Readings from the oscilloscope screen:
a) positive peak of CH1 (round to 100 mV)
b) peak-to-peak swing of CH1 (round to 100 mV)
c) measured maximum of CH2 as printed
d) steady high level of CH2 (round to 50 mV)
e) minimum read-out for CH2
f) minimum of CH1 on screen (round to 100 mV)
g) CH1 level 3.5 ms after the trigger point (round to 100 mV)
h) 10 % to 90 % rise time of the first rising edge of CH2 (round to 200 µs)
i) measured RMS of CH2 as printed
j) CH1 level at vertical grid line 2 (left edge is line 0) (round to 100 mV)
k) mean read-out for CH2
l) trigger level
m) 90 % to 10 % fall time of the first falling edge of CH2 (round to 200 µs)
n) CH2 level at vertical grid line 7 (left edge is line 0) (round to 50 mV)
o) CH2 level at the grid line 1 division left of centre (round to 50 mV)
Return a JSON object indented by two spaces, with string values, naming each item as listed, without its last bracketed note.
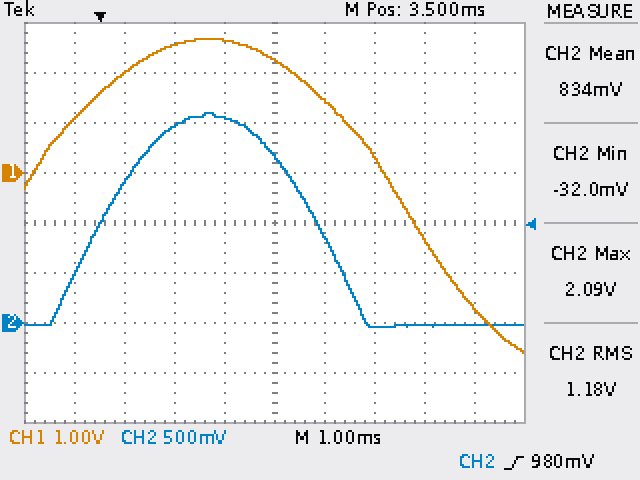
{
  "positive peak of CH1": "2.7 V",
  "peak-to-peak swing of CH1": "6.3 V",
  "measured maximum of CH2 as printed": "2.09 V",
  "steady high level of CH2": "2.05 V",
  "minimum read-out for CH2": "-32.0 mV",
  "minimum of CH1 on screen": "-3.6 V",
  "CH1 level 3.5 ms after the trigger point": "2.3 V",
  "10 % to 90 % rise time of the first rising edge of CH2": "2.0 ms",
  "measured RMS of CH2 as printed": "1.18 V",
  "CH1 level at vertical grid line 2 (left edge is line 0)": "2.0 V",
  "mean read-out for CH2": "834 mV",
  "trigger level": "980 mV",
  "90 % to 10 % fall time of the first falling edge of CH2": "2.0 ms",
  "CH2 level at vertical grid line 7 (left edge is line 0)": "-50 mV",
  "CH2 level at the grid line 1 division left of centre": "2.05 V"
}
